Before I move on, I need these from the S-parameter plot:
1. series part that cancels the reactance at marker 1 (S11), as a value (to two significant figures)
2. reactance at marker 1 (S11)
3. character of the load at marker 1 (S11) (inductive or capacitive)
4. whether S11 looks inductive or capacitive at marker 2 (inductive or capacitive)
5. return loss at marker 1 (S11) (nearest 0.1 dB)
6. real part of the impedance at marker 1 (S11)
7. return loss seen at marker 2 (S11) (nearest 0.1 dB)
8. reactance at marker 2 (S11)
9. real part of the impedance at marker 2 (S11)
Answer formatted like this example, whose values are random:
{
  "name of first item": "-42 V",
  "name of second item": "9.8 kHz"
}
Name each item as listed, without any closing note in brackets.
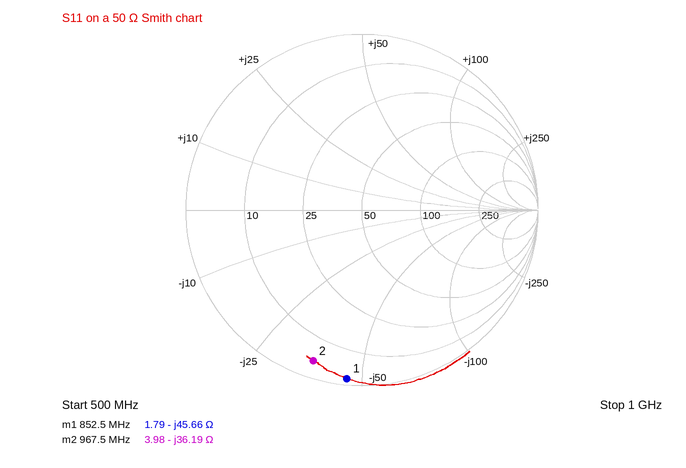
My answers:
{
  "series part that cancels the reactance at marker 1 (S11), as a value": "8.5 nH",
  "reactance at marker 1": "-45.66 Ω",
  "character of the load at marker 1 (S11)": "capacitive",
  "whether S11 looks inductive or capacitive at marker 2": "capacitive",
  "return loss at marker 1 (S11)": "0.3 dB",
  "real part of the impedance at marker 1": "1.79 Ω",
  "return loss seen at marker 2 (S11)": "0.9 dB",
  "reactance at marker 2": "-36.19 Ω",
  "real part of the impedance at marker 2": "3.98 Ω"
}
